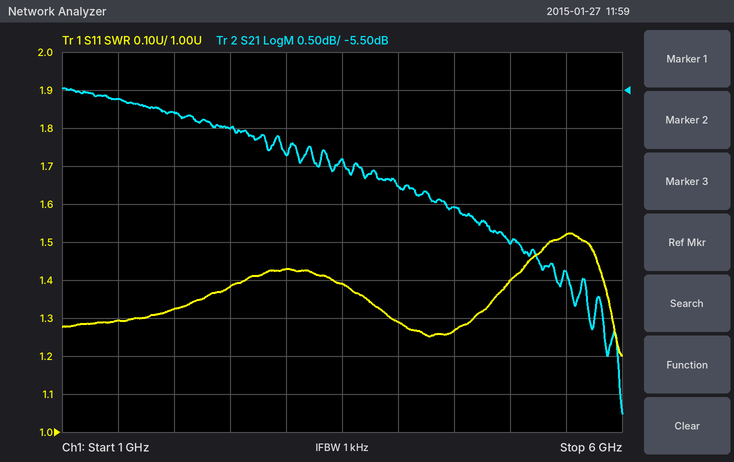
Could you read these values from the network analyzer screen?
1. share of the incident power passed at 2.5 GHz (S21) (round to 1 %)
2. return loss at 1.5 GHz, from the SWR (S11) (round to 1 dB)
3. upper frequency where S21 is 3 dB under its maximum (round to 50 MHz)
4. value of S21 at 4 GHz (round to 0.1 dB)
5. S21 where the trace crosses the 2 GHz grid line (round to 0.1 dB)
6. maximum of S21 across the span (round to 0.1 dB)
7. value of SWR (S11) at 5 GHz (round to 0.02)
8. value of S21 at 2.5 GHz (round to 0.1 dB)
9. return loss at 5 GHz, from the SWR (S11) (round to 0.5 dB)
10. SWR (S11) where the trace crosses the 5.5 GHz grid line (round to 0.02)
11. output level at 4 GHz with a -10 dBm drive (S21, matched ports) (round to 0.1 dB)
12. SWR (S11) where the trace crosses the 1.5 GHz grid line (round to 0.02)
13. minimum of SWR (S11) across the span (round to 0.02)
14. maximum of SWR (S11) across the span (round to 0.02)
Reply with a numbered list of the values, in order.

1. 25 %
2. 18 dB
3. 5.70 GHz
4. -6.8 dB
5. -5.8 dB
6. -5.5 dB
7. 1.40
8. -6.0 dB
9. 15.5 dB
10. 1.52
11. -16.8 dBm
12. 1.30
13. 1.20
14. 1.52
